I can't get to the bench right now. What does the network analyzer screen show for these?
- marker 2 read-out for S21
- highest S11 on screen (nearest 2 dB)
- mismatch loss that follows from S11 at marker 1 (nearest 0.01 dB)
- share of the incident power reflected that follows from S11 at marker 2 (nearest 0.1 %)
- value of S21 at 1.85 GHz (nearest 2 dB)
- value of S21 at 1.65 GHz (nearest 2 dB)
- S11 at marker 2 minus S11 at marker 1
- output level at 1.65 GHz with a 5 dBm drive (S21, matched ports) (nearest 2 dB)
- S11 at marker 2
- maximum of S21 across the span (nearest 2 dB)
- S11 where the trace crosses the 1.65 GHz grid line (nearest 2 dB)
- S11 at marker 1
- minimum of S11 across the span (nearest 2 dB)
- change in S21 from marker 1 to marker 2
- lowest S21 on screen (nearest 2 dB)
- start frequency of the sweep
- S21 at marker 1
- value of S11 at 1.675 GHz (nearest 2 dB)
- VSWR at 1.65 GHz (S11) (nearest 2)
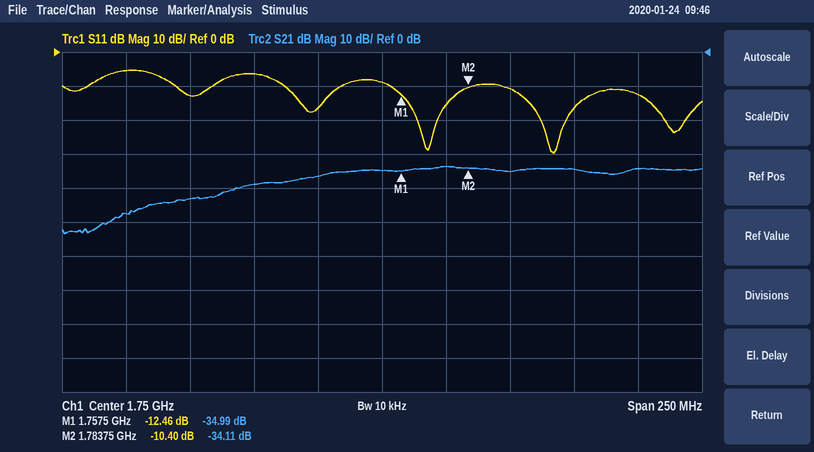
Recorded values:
-34.11 dB
-6 dB
0.25 dB
9.1 %
-34 dB
-48 dB
2.06 dB
-42 dBm
-10.40 dB
-34 dB
-6 dB
-12.46 dB
-30 dB
0.88 dB
-54 dB
1.625 GHz
-34.99 dB
-12 dB
4
